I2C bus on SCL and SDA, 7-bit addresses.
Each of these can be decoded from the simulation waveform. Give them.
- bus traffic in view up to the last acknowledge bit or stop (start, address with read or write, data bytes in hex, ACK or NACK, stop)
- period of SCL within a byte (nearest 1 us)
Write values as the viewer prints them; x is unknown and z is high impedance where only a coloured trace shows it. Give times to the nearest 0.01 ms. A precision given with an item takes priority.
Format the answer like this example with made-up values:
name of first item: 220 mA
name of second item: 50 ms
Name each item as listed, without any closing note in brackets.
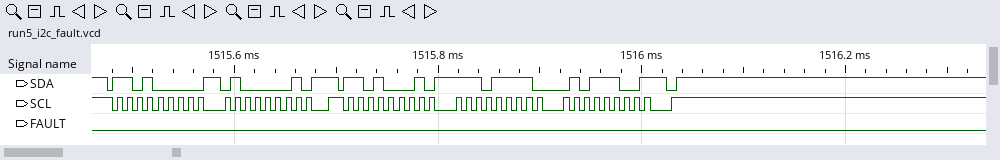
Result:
bus traffic in view up to the last acknowledge bit or stop: start, address 68 write ACK, 41 ACK, repeated start, address 68 read ACK, EF ACK, 5C NACK, stop
period of SCL within a byte: 10 us
